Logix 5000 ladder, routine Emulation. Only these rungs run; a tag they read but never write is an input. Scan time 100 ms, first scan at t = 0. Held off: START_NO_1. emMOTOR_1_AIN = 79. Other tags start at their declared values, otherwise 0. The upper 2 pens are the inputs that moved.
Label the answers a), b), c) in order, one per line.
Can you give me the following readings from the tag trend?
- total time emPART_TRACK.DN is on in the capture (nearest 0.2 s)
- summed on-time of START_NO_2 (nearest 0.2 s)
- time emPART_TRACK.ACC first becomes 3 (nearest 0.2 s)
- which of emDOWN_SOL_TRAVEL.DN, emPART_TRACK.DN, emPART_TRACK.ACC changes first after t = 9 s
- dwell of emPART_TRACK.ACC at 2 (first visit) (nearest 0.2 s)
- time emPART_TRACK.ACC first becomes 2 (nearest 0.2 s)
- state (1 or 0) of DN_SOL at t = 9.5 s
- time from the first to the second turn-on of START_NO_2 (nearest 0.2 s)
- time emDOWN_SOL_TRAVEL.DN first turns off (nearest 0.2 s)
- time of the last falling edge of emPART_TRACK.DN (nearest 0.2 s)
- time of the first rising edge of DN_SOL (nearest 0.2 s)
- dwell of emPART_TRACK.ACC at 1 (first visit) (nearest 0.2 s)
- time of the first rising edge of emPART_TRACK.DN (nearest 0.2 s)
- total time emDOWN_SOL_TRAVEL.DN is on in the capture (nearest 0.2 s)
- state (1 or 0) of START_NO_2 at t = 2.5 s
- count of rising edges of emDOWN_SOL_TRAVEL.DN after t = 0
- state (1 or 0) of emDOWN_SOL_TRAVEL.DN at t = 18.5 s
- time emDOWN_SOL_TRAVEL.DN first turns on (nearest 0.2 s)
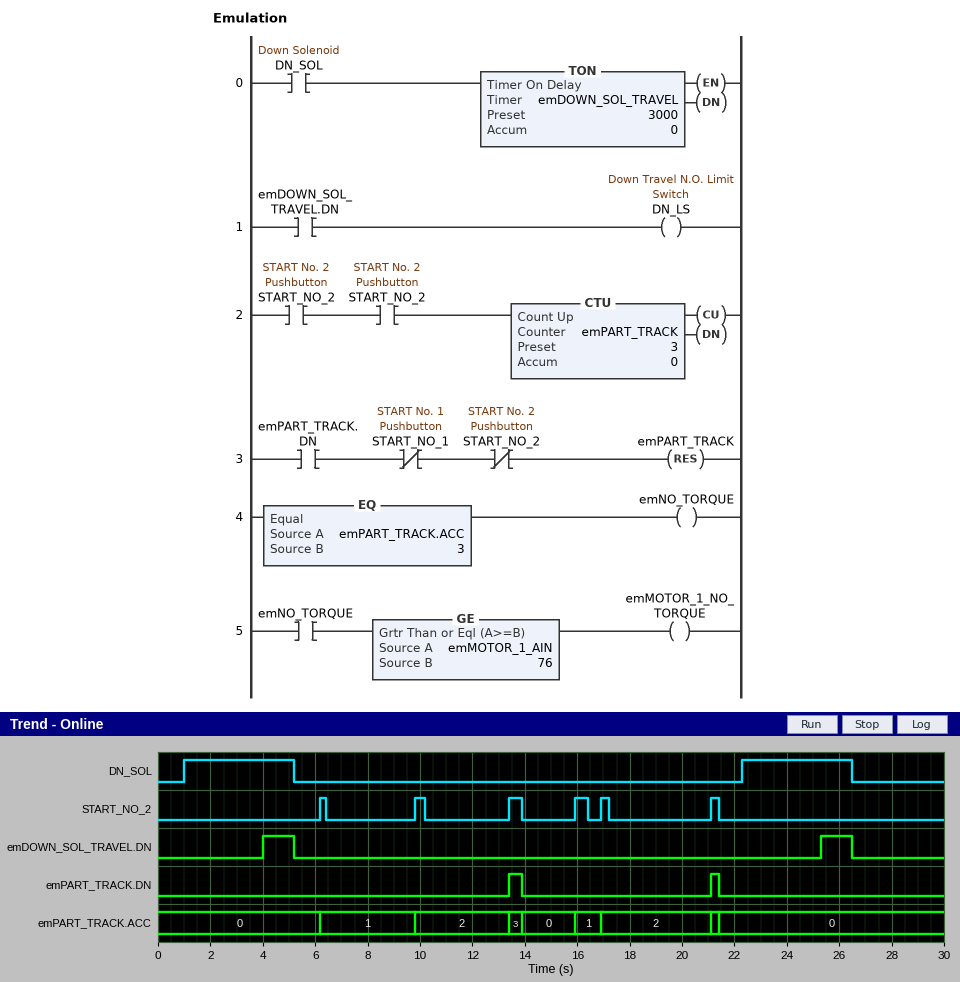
a) 0.8 s
b) 2.2 s
c) 13.4 s
d) emPART_TRACK.ACC
e) 3.6 s
f) 9.8 s
g) 0
h) 3.6 s
i) 5.2 s
j) 21.4 s
k) 1.0 s
l) 3.6 s
m) 13.4 s
n) 2.4 s
o) 0
p) 2
q) 0
r) 4.0 s
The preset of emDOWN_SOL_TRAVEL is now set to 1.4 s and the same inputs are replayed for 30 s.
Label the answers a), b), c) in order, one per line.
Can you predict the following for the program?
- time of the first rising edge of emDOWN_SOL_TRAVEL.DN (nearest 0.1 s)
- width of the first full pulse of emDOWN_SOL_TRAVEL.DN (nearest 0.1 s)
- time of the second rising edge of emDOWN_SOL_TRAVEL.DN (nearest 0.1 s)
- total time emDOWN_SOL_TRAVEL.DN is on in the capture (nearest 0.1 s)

a) 2.4 s
b) 2.8 s
c) 23.7 s
d) 5.6 s
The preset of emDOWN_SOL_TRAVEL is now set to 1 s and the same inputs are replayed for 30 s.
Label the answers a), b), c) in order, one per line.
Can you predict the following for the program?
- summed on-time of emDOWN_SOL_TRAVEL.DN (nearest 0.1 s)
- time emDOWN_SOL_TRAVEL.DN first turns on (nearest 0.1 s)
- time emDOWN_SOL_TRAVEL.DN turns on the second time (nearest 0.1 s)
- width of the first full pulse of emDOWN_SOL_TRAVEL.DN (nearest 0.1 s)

a) 6.4 s
b) 2.0 s
c) 23.3 s
d) 3.2 s
